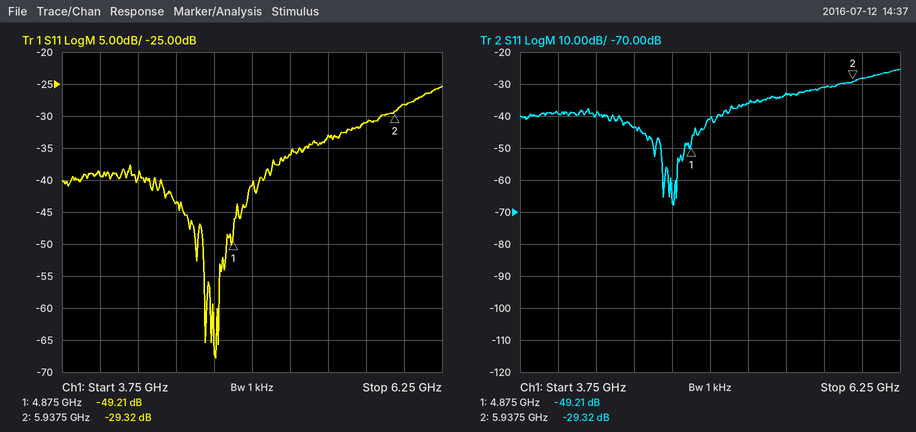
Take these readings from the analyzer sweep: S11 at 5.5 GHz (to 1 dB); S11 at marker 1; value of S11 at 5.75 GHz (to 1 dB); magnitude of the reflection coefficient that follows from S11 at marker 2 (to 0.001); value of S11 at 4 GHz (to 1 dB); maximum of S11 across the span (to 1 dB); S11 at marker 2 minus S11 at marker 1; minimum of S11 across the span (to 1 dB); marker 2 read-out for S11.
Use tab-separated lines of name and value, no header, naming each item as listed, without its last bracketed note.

S11 at 5.5 GHz	-33 dB
S11 at marker 1	-49.21 dB
value of S11 at 5.75 GHz	-31 dB
magnitude of the reflection coefficient that follows from S11 at marker 2	0.034
value of S11 at 4 GHz	-39 dB
maximum of S11 across the span	-25 dB
S11 at marker 2 minus S11 at marker 1	19.89 dB
minimum of S11 across the span	-68 dB
marker 2 read-out for S11	-29.32 dB
